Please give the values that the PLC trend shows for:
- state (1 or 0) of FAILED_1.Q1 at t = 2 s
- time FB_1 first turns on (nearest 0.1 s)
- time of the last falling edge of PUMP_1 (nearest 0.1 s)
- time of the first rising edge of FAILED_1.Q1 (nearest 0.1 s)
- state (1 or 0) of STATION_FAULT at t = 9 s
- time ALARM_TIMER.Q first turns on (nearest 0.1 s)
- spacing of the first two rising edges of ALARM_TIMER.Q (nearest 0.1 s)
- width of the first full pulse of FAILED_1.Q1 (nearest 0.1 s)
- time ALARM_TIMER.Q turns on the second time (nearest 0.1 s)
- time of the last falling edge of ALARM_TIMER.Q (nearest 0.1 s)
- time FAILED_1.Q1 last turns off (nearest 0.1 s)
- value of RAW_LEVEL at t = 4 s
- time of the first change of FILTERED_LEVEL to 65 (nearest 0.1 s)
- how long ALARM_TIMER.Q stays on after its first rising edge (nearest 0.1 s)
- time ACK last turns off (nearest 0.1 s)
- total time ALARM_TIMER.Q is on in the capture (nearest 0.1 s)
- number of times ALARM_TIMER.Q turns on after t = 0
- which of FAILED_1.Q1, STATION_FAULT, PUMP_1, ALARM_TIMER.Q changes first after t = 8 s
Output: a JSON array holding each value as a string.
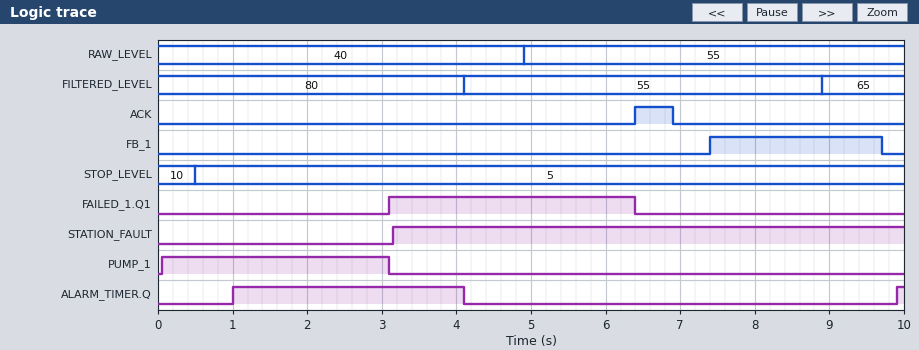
["0", "7.4 s", "3.1 s", "3.1 s", "1", "1.0 s", "8.9 s", "3.3 s", "9.9 s", "4.1 s", "6.4 s", "40", "8.9 s", "3.1 s", "6.9 s", "3.2 s", "2", "ALARM_TIMER.Q"]
